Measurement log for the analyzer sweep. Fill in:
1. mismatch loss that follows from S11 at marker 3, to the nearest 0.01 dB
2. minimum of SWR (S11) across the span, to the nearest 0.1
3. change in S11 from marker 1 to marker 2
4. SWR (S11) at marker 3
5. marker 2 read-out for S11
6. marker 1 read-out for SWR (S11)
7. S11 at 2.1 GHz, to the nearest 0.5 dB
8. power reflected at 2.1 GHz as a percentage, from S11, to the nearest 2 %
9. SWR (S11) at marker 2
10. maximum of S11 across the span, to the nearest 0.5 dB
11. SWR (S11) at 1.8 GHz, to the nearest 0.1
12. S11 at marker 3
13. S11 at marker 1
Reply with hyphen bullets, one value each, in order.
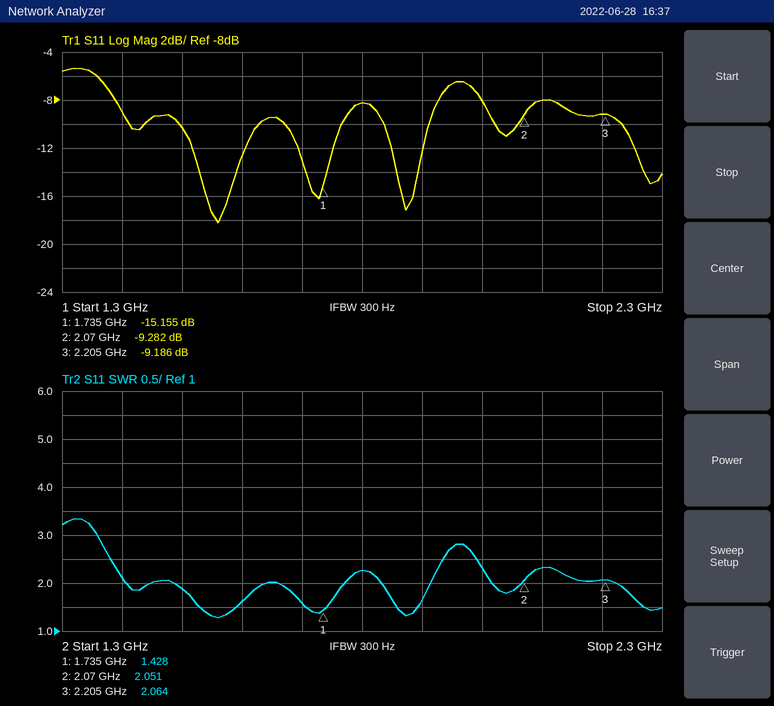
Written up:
- 0.56 dB
- 1.3
- 5.873 dB
- 2.064
- -9.282 dB
- 1.428
- -8.0 dB
- 16 %
- 2.051
- -5.5 dB
- 2.3
- -9.186 dB
- -15.155 dB
